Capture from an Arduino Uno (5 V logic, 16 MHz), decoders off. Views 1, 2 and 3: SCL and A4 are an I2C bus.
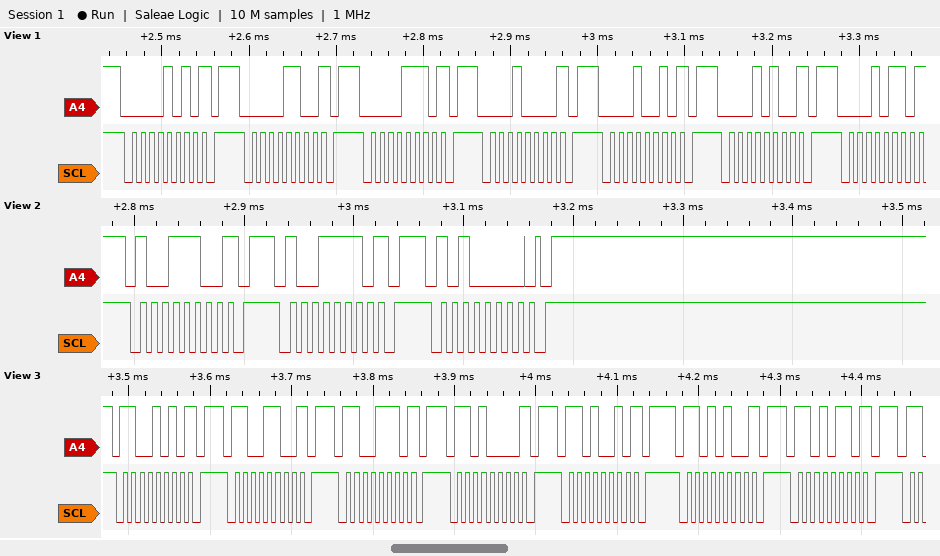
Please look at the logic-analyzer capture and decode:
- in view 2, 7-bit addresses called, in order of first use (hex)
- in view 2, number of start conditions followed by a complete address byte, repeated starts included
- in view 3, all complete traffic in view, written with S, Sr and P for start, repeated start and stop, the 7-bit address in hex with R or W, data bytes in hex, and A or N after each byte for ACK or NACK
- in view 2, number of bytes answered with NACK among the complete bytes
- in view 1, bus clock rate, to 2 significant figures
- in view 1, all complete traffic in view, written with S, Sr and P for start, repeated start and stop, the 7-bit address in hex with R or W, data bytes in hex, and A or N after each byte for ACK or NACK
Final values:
0x4E 0x4F 0x50
3
S 65W N P S 66W N P S 67W N P S 68W N P S 69W N P S 6AW N P S 6BW N P
2
100 kHz
S 05W N P S 06W N P S 07W N P S 08W N P S 09W N P S 0AW N P S 0BW N
